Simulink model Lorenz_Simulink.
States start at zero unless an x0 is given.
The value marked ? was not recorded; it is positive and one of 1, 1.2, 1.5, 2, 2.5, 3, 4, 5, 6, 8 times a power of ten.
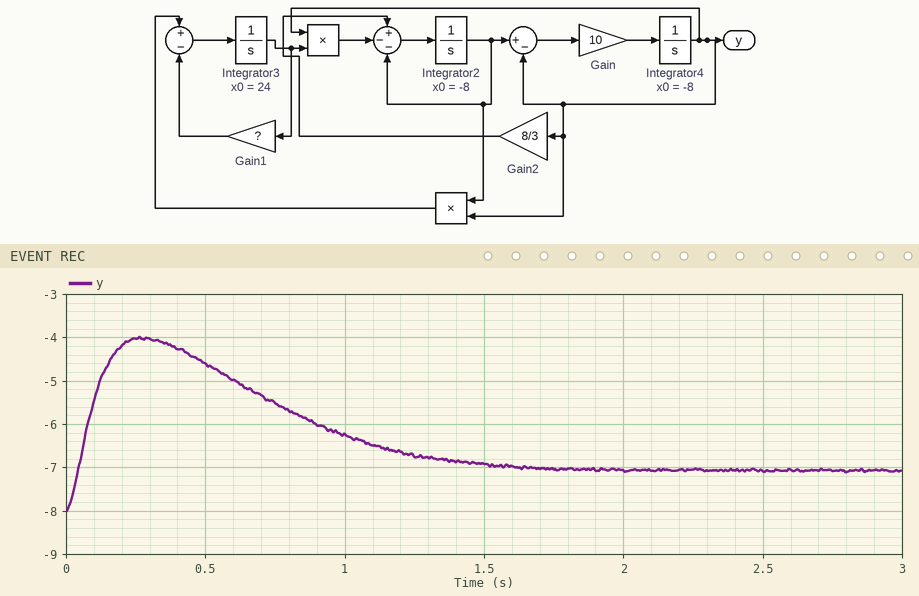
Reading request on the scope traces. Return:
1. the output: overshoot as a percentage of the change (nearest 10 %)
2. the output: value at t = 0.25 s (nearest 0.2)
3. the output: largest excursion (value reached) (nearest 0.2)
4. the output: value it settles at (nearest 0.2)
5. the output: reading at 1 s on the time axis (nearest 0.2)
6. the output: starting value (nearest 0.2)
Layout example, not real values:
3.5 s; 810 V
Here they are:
330 %; -4.0; -4.0; -7.0; -6.2; -8.0
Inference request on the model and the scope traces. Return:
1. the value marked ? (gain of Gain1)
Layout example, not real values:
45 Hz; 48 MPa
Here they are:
30
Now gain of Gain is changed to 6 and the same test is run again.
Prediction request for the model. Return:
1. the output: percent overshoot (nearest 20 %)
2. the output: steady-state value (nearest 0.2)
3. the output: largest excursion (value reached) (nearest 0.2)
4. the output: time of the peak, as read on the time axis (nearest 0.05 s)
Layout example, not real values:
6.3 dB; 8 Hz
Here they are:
280 %; -7.0; -4.4; 0.35 s
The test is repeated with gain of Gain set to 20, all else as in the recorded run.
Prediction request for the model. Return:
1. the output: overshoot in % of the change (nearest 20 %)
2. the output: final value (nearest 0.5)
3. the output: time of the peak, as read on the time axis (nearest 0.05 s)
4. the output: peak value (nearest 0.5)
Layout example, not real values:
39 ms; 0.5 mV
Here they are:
360 %; -7.0; 0.20 s; -3.5
